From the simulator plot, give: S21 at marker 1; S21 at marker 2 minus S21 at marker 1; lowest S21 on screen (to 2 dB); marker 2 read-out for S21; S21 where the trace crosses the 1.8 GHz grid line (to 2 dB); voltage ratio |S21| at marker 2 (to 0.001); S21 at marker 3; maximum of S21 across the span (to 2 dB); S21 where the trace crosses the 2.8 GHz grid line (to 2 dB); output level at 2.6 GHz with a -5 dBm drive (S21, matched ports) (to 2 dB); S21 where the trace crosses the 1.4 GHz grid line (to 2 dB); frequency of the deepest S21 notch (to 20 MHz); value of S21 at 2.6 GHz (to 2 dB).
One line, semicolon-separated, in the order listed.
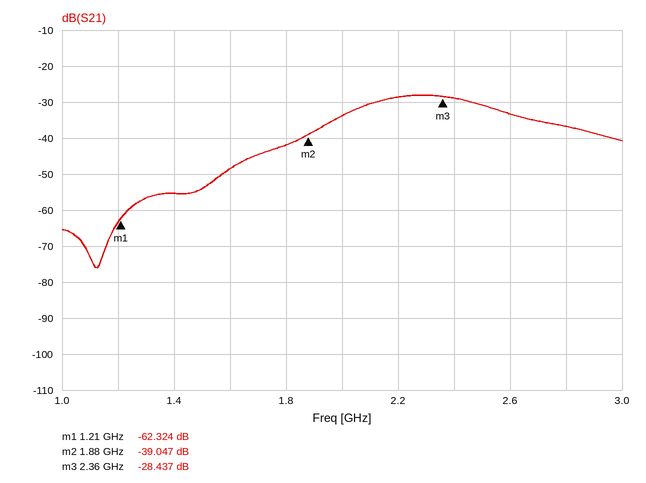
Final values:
-62.324 dB; 23.277 dB; -76 dB; -39.047 dB; -42 dB; 0.011; -28.437 dB; -28 dB; -36 dB; -38 dBm; -56 dB; 1.12 GHz; -34 dB
